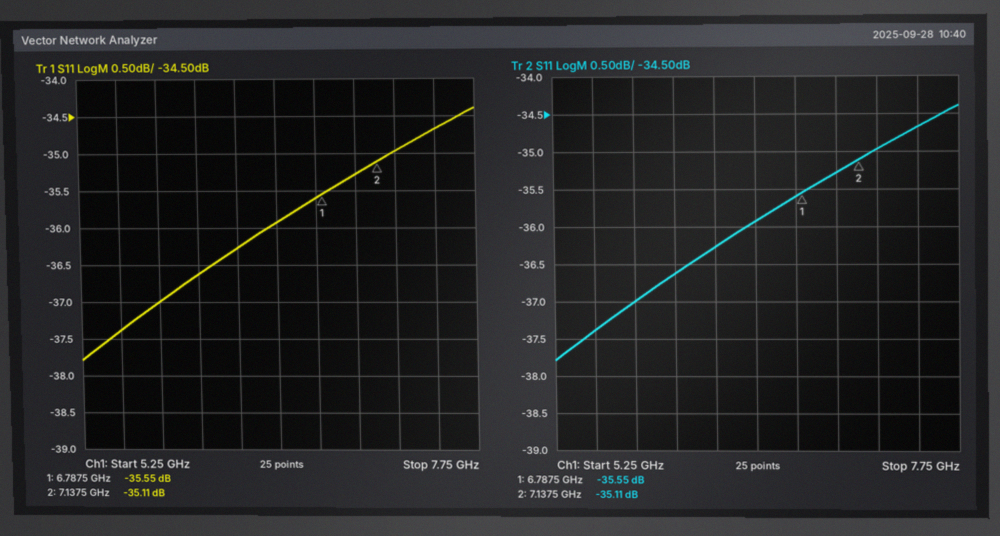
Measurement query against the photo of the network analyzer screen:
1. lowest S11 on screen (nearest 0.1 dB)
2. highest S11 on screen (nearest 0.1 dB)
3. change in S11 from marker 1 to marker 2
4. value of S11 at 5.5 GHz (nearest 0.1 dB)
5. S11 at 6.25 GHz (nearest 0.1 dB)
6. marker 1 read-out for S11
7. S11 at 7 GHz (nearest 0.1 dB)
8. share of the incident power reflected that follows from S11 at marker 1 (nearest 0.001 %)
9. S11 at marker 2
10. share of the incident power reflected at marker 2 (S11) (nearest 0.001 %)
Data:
-37.8 dB
-34.4 dB
0.44 dB
-37.4 dB
-36.3 dB
-35.55 dB
-35.3 dB
0.028 %
-35.11 dB
0.031 %
